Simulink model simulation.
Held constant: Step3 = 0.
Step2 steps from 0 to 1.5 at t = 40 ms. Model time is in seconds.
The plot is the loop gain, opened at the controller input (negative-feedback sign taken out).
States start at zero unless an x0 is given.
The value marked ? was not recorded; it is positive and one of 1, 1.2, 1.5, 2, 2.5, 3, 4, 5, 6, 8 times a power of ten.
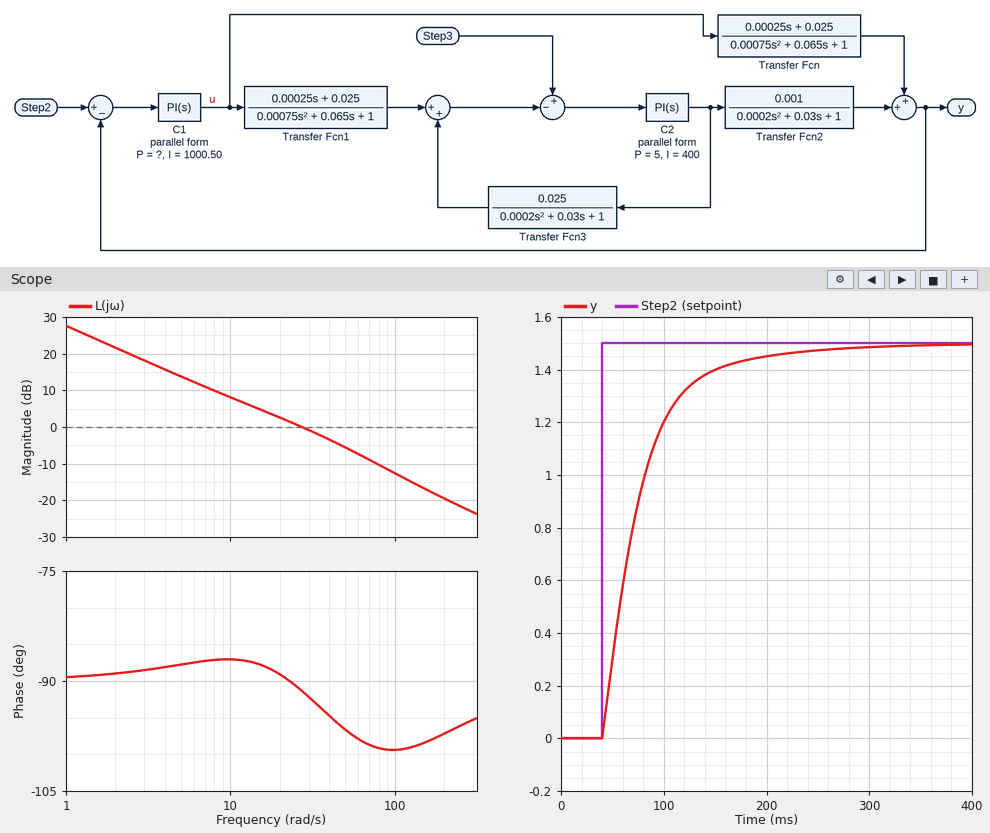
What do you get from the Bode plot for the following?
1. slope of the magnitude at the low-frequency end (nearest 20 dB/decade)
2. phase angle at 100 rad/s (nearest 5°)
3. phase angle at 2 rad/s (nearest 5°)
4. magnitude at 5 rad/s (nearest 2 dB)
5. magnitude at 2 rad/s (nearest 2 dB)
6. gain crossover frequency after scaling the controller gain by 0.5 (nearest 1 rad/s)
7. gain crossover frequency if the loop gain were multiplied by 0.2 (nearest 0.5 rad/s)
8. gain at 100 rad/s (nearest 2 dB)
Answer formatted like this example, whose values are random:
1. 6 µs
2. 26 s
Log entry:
1. -20 dB/decade
2. -100°
3. -90°
4. 14 dB
5. 22 dB
6. 13 rad/s
7. 5.0 rad/s
8. -12 dB
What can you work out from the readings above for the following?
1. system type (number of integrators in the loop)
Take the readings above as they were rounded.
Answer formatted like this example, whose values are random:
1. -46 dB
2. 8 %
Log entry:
1. 1
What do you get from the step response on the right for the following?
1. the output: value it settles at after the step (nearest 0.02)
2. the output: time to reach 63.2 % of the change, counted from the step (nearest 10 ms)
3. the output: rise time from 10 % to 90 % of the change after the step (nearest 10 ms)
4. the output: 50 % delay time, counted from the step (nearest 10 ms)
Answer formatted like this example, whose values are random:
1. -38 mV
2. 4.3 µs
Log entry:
1. 1.50
2. 40 ms
3. 80 ms
4. 30 ms
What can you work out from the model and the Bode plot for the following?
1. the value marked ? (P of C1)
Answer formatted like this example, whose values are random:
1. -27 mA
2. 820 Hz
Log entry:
1. 60
